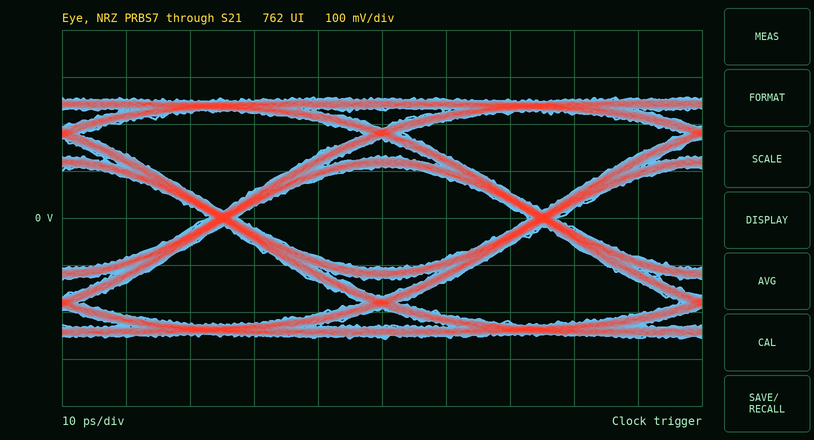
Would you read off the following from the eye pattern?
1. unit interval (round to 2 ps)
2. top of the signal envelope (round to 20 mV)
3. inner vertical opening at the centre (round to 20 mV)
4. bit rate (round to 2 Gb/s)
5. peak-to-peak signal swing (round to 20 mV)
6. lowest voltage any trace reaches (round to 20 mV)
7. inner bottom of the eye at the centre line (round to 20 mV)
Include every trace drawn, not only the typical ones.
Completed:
50 ps
260 mV
220 mV
20 Gb/s
520 mV
-260 mV
-100 mV
